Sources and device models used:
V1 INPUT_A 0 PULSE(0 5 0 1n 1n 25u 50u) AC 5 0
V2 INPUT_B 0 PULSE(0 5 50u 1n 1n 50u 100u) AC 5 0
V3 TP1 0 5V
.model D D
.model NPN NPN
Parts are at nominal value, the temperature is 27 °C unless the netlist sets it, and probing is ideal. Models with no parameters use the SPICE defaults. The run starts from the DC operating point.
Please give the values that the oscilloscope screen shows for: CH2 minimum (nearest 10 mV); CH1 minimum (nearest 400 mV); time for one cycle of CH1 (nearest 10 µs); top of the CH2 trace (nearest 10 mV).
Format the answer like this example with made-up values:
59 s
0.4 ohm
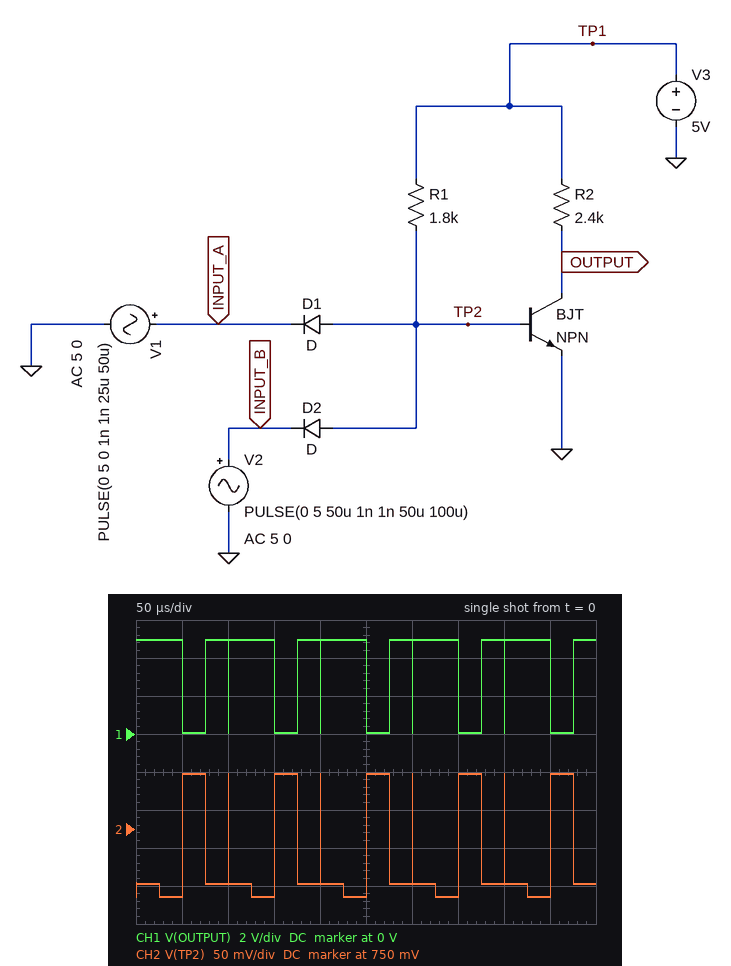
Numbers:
660 mV
0 V
100 µs
820 mV
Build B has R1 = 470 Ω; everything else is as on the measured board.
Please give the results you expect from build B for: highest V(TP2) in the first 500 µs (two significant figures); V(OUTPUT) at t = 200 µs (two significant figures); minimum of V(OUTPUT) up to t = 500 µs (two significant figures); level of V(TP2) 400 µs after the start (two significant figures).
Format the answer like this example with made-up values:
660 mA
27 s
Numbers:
850 mV
4.8 V
21 mV
710 mV
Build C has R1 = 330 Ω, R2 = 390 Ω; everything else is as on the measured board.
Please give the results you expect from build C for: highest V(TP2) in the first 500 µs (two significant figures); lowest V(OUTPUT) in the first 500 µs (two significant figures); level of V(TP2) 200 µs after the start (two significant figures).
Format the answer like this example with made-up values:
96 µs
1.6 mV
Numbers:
870 mV
29 mV
720 mV
